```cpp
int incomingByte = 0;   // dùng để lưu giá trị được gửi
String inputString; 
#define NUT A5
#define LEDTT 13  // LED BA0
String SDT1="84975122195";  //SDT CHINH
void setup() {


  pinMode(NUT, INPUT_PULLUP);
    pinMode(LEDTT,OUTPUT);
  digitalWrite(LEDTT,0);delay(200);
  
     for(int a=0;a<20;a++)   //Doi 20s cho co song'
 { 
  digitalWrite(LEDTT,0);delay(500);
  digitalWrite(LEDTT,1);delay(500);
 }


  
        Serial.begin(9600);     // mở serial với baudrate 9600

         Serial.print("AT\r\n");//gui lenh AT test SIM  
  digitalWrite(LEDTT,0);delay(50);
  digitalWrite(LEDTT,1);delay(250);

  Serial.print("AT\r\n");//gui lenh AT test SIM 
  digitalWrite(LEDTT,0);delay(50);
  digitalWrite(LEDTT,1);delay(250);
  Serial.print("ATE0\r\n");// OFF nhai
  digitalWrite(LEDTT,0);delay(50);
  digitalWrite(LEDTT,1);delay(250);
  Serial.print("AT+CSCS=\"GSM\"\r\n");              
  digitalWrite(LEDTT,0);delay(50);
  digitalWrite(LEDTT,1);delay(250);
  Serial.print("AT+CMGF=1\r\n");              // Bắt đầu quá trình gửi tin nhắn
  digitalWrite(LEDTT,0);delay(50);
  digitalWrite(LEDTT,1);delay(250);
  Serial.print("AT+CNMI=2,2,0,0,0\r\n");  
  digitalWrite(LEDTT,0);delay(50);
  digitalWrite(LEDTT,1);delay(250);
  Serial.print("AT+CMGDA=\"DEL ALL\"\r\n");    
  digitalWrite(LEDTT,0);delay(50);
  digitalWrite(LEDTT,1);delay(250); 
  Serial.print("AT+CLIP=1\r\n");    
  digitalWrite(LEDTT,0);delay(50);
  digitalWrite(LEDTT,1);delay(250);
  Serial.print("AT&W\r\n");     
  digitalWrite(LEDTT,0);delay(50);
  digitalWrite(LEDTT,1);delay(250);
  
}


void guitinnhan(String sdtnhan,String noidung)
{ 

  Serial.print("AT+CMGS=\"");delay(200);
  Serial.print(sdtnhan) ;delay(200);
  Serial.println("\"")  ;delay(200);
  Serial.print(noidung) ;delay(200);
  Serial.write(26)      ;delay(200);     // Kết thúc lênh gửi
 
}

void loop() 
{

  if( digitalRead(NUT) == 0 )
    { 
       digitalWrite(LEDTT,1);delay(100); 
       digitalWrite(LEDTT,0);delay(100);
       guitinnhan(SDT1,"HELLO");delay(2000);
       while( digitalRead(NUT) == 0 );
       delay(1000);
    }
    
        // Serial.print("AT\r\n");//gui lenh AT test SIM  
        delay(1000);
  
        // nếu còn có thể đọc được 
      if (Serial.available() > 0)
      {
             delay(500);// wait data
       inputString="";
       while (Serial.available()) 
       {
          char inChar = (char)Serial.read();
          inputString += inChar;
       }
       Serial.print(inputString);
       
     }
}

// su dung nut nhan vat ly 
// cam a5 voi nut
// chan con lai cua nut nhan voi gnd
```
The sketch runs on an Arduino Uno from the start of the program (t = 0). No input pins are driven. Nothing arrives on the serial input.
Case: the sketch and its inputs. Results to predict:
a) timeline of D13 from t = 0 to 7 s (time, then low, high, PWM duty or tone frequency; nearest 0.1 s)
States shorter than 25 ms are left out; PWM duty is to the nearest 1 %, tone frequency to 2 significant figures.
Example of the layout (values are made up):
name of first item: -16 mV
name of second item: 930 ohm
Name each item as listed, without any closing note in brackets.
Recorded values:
timeline of D13 from t = 0 to 7 s: 0 s low; 0.7 s high; 1.2 s low; 1.7 s high; 2.2 s low; 2.7 s high; 3.2 s low; 3.7 s high; 4.2 s low; 4.7 s high; 5.2 s low; 5.7 s high; 6.2 s low; 6.7 s high
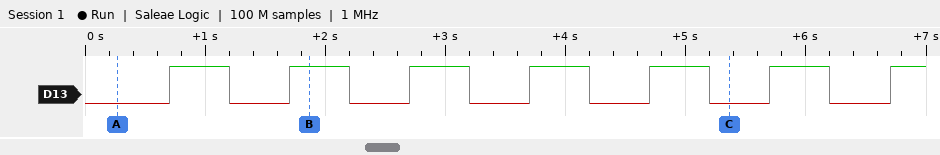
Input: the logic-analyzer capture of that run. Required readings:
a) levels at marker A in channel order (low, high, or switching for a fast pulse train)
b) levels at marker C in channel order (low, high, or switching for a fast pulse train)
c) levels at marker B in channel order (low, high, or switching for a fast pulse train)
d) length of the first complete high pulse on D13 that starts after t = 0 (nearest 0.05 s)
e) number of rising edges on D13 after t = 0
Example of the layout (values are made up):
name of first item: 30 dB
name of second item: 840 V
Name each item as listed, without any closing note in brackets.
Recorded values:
levels at marker A in channel order: D13 low
levels at marker C in channel order: D13 low
levels at marker B in channel order: D13 high
length of the first complete high pulse on D13 that starts after t = 0: 0.50 s
number of rising edges on D13 after t = 0: 7
